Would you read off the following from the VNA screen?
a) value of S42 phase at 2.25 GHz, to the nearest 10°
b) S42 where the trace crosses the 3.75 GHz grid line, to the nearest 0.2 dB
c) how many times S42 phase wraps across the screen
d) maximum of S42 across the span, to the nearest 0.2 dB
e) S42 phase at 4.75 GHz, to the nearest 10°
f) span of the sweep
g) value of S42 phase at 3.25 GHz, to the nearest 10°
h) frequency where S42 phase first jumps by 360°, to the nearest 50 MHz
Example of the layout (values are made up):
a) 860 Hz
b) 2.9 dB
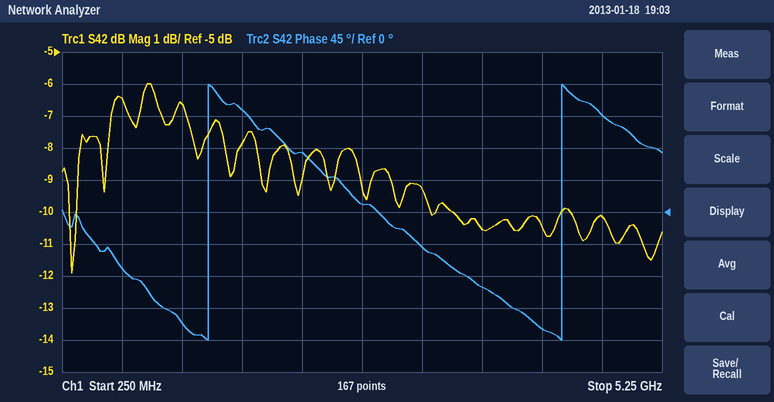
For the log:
a) 80°
b) -10.6 dB
c) 2
d) -6.0 dB
e) 140°
f) 5 GHz
g) -50°
h) 1.45 GHz
